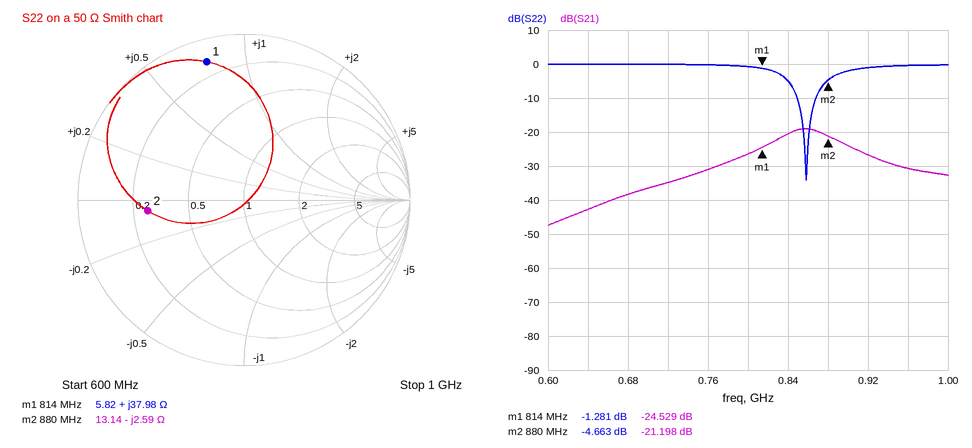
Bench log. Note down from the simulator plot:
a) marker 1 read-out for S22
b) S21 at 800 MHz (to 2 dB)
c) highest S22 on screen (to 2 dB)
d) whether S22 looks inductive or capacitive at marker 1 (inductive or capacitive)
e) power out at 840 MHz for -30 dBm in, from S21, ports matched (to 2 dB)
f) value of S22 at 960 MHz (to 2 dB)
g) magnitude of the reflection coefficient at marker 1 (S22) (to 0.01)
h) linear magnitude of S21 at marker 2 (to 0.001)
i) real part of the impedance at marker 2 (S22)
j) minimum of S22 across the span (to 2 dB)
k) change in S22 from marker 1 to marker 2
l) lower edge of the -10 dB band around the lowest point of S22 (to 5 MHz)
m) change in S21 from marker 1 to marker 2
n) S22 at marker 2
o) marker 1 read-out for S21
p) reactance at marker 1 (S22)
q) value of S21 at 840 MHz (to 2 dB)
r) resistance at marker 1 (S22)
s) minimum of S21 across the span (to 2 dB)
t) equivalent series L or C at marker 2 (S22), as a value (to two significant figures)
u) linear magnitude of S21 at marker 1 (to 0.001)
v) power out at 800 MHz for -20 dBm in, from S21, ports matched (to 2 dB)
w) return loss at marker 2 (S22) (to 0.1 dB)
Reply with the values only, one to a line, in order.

-1.281 dB
-26 dB
0 dB
inductive
-50 dBm
0 dB
0.86
0.087
13.14 Ω
-34 dB
-3.382 dB
850 MHz
3.331 dB
-4.663 dB
-24.529 dB
+37.98 Ω
-20 dB
5.82 Ω
-48 dB
70 pF
0.059
-46 dBm
4.7 dB
